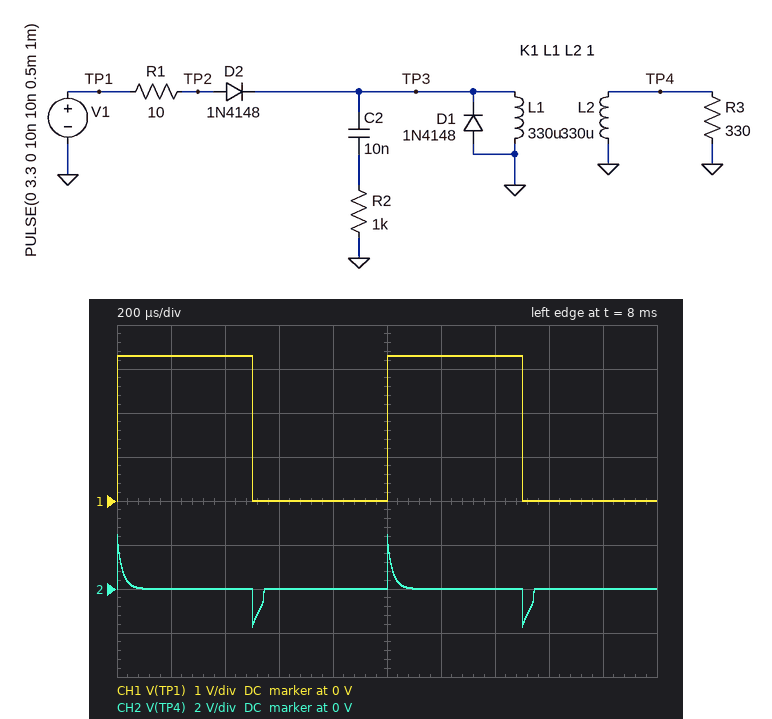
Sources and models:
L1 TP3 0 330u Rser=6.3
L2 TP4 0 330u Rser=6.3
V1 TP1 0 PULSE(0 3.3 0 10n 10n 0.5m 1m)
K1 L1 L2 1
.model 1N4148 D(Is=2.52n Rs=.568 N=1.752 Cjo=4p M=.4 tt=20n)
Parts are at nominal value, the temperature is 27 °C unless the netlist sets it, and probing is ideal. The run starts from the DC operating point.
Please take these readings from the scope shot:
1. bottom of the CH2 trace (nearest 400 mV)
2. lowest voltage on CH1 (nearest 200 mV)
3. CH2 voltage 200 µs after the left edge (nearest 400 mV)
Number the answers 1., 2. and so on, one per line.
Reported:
1. -1.6 V
2. 0 V
3. 0 V
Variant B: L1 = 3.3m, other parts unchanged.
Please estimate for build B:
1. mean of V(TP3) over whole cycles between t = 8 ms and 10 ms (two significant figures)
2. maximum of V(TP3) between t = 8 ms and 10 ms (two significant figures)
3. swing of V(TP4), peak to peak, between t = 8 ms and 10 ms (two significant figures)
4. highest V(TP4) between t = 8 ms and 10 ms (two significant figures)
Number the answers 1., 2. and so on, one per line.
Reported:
1. 440 mV
2. 2.7 V
3. 1.4 V
4. 830 mV
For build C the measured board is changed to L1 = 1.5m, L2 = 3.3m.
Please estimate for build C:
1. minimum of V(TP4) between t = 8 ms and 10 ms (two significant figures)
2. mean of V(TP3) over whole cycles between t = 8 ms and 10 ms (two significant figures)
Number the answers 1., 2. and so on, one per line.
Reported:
1. -2.5 V
2. 450 mV
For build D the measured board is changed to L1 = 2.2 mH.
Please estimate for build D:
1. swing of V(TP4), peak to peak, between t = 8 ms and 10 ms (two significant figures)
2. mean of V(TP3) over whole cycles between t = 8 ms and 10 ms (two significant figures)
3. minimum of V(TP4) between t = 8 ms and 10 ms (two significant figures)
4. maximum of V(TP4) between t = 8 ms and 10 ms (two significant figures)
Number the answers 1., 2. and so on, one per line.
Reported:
1. 1.7 V
2. 450 mV
3. -680 mV
4. 1.0 V
